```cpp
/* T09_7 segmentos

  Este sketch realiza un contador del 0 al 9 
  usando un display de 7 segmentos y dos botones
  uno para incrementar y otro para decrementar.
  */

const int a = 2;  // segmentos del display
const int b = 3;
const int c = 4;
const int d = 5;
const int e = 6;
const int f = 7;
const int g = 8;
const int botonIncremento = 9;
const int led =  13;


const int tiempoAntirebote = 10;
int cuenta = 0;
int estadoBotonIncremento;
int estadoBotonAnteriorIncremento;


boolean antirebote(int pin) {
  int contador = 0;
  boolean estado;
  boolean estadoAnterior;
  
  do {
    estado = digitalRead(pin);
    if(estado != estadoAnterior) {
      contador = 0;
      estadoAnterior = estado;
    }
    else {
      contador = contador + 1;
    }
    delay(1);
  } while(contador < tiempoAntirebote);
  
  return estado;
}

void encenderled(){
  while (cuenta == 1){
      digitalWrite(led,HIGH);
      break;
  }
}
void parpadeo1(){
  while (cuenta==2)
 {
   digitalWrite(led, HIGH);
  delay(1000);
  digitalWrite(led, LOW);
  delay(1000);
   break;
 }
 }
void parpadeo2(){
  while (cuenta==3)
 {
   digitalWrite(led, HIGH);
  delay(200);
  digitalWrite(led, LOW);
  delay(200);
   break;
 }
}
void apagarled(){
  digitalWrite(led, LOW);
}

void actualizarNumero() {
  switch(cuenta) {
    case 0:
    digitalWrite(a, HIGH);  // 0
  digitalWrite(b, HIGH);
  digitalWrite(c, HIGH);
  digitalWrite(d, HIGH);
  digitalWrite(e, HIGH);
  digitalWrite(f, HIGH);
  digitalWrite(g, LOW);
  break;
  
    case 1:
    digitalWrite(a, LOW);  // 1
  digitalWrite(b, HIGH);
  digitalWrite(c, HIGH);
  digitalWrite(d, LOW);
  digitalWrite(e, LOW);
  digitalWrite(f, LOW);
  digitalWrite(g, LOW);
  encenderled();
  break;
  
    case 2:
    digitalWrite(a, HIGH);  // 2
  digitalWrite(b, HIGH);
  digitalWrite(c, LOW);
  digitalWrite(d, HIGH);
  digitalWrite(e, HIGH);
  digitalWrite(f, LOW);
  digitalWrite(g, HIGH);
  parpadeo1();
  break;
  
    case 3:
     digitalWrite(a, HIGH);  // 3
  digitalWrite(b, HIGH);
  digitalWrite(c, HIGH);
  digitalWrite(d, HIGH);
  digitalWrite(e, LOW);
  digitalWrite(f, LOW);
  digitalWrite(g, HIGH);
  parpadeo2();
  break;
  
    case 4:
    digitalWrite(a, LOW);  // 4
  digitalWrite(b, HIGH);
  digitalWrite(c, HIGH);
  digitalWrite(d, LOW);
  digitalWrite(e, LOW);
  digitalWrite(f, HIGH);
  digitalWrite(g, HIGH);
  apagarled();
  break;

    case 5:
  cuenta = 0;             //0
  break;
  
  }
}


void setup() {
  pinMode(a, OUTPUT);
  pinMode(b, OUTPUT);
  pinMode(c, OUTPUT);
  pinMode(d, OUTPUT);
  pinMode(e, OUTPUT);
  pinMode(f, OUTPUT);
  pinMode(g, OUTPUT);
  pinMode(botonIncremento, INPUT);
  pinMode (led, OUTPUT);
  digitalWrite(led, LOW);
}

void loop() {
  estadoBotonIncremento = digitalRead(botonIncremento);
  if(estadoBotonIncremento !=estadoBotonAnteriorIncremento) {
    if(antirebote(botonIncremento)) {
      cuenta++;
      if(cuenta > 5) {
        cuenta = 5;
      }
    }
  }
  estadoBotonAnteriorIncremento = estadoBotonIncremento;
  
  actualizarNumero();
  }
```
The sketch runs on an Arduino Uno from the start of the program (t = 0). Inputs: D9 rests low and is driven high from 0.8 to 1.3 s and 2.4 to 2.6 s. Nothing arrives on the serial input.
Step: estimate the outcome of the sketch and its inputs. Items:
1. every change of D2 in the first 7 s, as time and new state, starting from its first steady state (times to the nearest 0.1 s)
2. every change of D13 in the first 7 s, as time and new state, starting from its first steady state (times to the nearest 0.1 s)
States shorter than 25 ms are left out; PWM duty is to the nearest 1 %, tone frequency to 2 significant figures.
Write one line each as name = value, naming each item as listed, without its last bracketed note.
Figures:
every change of D2 in the first 7 s, as time and new state, starting from its first steady state = 0 s high; 0.8 s low; 2.4 s high
every change of D13 in the first 7 s, as time and new state, starting from its first steady state = 0 s low; 0.8 s high; 3.4 s low; 4.4 s high; 5.4 s low; 6.4 s high
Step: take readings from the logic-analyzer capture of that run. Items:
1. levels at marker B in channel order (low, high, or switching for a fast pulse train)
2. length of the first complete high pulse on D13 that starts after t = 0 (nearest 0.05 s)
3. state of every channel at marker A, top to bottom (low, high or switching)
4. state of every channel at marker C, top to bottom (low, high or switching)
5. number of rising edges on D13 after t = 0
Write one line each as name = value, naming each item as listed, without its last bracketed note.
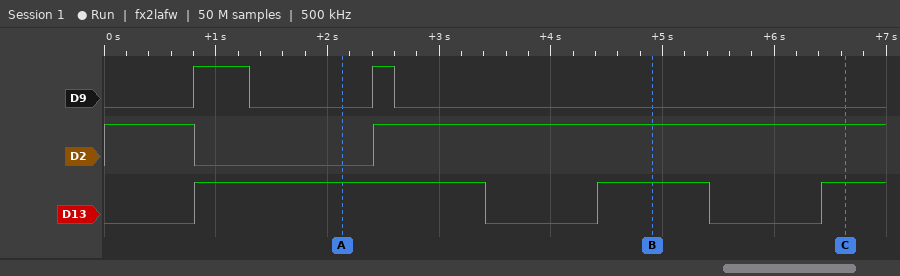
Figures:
levels at marker B in channel order = D9 low, D2 high, D13 high
length of the first complete high pulse on D13 that starts after t = 0 = 2.60 s
state of every channel at marker A, top to bottom = D9 low, D2 low, D13 high
state of every channel at marker C, top to bottom = D9 low, D2 high, D13 high
number of rising edges on D13 after t = 0 = 3
